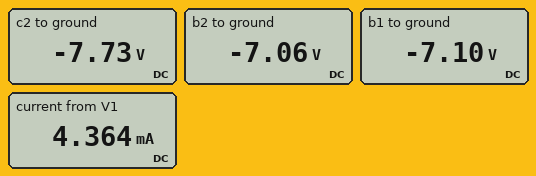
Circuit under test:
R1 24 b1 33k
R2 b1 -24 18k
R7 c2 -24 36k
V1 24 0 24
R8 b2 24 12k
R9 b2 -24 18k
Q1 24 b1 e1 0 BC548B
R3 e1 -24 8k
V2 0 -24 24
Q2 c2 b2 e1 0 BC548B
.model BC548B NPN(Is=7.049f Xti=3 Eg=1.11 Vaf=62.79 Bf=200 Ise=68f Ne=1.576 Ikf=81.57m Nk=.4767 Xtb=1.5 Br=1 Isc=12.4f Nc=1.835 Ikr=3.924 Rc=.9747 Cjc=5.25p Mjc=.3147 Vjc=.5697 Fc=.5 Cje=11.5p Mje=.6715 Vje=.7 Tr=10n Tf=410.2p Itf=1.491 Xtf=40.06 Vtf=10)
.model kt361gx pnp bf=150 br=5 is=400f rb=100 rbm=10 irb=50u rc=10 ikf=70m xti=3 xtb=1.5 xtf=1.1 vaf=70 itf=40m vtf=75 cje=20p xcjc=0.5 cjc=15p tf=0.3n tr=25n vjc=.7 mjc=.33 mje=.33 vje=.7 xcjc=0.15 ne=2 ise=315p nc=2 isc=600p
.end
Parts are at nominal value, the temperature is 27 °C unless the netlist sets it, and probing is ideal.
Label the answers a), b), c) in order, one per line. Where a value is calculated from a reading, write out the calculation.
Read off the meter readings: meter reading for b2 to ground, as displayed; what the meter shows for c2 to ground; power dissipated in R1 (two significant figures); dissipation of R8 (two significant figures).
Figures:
a) -7.06 V
b) -7.73 V
c) (24 V - (-7.1 V))^2 / 33 kΩ = 29 mW
d) (24 V - (-7.06 V))^2 / 12 kΩ = 80 mW
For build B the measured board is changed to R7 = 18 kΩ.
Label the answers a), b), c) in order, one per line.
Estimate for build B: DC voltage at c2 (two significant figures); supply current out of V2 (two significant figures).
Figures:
a) -7.8 V
b) 4.8 mA
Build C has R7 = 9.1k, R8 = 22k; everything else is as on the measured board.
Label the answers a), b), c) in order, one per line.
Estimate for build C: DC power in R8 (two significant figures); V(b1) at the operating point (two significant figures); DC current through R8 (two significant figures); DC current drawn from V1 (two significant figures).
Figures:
a) 52 mW
b) -7.2 V
c) 1.5 mA
d) 5.2 mA
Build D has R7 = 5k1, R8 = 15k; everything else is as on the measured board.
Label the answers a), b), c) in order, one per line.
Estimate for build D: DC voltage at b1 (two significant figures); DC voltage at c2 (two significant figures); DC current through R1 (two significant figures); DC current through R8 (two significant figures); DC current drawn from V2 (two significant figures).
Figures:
a) -7.2 V
b) -9.9 V
c) 950 µA
d) 2.2 mA
e) 6.5 mA
